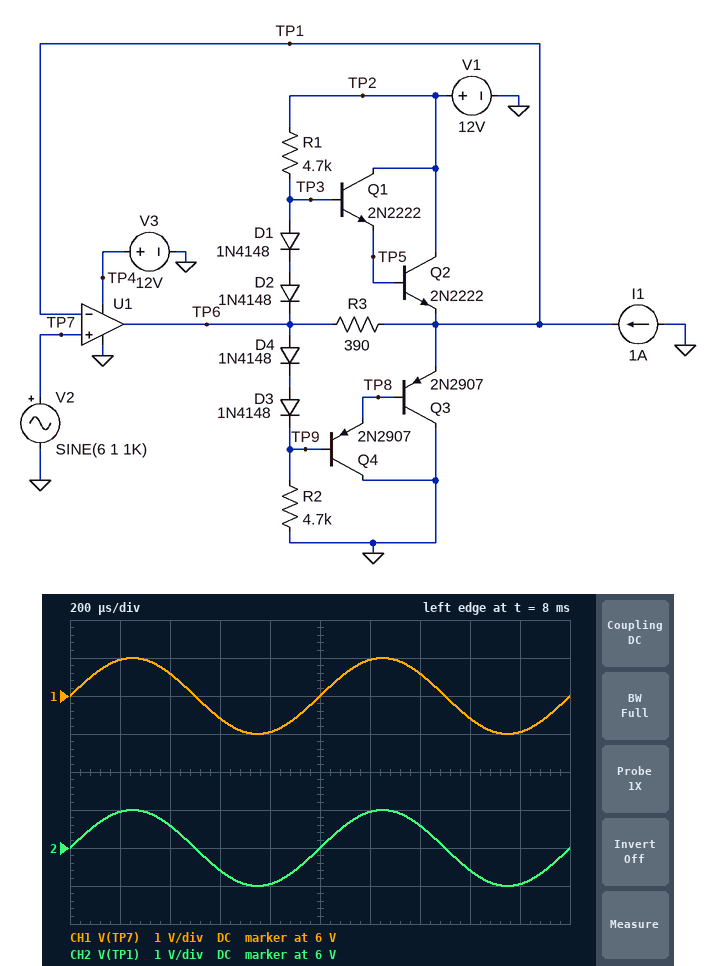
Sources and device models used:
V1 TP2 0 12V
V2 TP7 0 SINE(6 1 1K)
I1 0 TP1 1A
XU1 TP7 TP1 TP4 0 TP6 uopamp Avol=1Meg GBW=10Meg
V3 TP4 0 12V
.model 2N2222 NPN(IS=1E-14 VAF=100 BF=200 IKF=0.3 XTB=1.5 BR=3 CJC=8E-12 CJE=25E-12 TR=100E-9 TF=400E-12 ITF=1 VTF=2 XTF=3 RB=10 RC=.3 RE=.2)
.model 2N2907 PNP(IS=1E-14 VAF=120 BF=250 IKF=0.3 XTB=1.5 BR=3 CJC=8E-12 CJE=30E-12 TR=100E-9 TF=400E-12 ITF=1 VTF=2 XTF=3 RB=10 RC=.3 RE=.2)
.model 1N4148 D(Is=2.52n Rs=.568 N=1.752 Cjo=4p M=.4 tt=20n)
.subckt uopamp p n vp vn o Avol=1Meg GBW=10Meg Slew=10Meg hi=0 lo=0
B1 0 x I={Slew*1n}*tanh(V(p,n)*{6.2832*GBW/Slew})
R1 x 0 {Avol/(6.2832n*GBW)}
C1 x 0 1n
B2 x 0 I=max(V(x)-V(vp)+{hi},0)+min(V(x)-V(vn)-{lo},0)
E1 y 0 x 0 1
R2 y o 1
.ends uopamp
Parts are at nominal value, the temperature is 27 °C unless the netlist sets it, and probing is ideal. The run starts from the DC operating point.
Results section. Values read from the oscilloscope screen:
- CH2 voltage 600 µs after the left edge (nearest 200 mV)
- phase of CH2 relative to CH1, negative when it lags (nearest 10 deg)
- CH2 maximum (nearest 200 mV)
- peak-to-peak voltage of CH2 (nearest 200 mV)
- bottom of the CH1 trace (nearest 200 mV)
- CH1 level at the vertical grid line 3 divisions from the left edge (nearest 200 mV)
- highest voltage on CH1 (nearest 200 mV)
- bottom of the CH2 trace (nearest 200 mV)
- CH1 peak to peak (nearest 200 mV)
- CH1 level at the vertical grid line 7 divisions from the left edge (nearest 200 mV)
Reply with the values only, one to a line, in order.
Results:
5.4 V
0 deg
7.0 V
2.0 V
5.0 V
5.4 V
7.0 V
5.0 V
2.0 V
6.6 V
